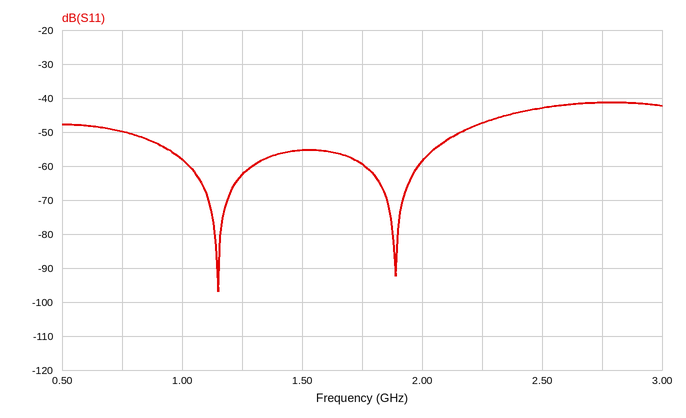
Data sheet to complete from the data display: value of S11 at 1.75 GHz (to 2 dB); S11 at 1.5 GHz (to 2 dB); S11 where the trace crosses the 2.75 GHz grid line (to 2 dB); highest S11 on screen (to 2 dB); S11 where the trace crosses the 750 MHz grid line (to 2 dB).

-60 dB
-56 dB
-42 dB
-42 dB
-50 dB
